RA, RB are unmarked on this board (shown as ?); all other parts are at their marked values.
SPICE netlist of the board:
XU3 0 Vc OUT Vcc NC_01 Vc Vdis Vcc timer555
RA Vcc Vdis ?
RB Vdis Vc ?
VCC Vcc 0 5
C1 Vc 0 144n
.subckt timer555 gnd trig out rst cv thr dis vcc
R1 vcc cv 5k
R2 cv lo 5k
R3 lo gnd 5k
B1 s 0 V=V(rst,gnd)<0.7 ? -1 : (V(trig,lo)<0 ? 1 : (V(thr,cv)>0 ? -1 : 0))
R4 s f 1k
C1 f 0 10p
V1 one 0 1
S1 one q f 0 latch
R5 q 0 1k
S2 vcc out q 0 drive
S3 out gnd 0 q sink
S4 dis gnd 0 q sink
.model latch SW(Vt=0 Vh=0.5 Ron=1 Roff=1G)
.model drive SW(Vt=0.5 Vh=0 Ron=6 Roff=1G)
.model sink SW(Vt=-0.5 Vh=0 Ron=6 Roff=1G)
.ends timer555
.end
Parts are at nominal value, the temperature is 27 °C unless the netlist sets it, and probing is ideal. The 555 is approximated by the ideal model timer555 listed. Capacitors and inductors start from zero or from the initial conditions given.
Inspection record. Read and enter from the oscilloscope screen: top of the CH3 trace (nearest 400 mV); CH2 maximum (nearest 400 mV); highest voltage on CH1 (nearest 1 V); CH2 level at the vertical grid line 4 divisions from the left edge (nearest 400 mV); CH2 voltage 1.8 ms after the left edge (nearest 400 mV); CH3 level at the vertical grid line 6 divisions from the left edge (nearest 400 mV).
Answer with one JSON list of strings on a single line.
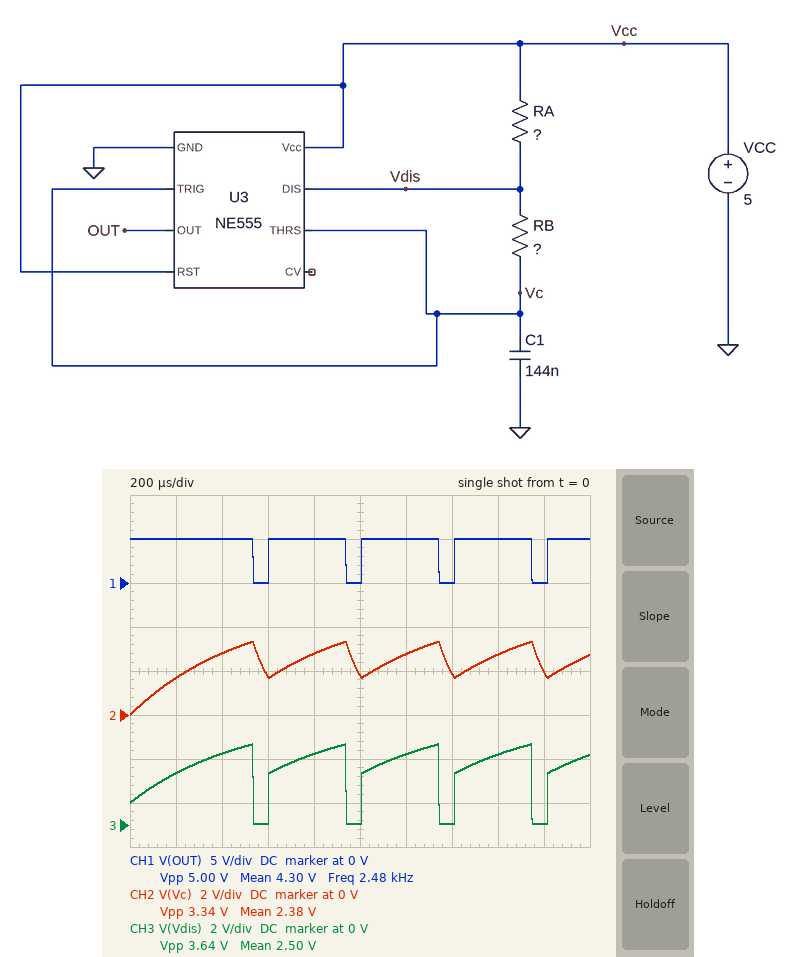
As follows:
["3.6 V", "3.2 V", "5 V", "2.8 V", "2.0 V", "3.2 V"]
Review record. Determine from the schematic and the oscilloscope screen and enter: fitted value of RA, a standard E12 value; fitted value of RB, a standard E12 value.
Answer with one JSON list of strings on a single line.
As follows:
["2.7 kΩ", "680 Ω"]
